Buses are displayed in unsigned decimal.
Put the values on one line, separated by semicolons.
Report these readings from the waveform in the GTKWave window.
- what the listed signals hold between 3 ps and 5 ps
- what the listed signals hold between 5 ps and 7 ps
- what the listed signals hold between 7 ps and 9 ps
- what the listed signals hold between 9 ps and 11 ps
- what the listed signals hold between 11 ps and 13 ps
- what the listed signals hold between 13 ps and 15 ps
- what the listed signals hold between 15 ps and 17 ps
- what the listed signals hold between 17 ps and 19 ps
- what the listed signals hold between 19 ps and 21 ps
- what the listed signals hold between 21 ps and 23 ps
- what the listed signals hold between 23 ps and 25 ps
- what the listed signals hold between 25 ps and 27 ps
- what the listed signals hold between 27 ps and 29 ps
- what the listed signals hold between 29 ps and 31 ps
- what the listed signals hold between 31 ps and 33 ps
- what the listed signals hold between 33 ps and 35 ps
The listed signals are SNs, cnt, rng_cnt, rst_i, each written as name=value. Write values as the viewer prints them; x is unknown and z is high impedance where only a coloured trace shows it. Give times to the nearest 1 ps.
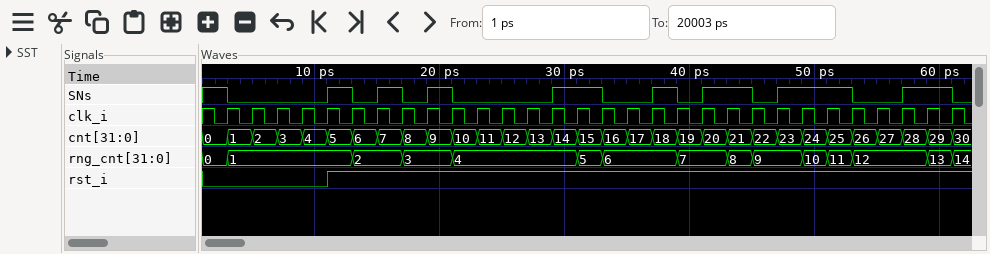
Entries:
SNs=0, cnt=1, rng_cnt=1, rst_i=0; SNs=0, cnt=2, rng_cnt=1, rst_i=0; SNs=0, cnt=3, rng_cnt=1, rst_i=0; SNs=0, cnt=4, rng_cnt=1, rst_i=0; SNs=1, cnt=5, rng_cnt=1, rst_i=1; SNs=0, cnt=6, rng_cnt=2, rst_i=1; SNs=1, cnt=7, rng_cnt=2, rst_i=1; SNs=0, cnt=8, rng_cnt=3, rst_i=1; SNs=1, cnt=9, rng_cnt=3, rst_i=1; SNs=0, cnt=10, rng_cnt=4, rst_i=1; SNs=0, cnt=11, rng_cnt=4, rst_i=1; SNs=0, cnt=12, rng_cnt=4, rst_i=1; SNs=0, cnt=13, rng_cnt=4, rst_i=1; SNs=1, cnt=14, rng_cnt=4, rst_i=1; SNs=1, cnt=15, rng_cnt=5, rst_i=1; SNs=0, cnt=16, rng_cnt=6, rst_i=1
